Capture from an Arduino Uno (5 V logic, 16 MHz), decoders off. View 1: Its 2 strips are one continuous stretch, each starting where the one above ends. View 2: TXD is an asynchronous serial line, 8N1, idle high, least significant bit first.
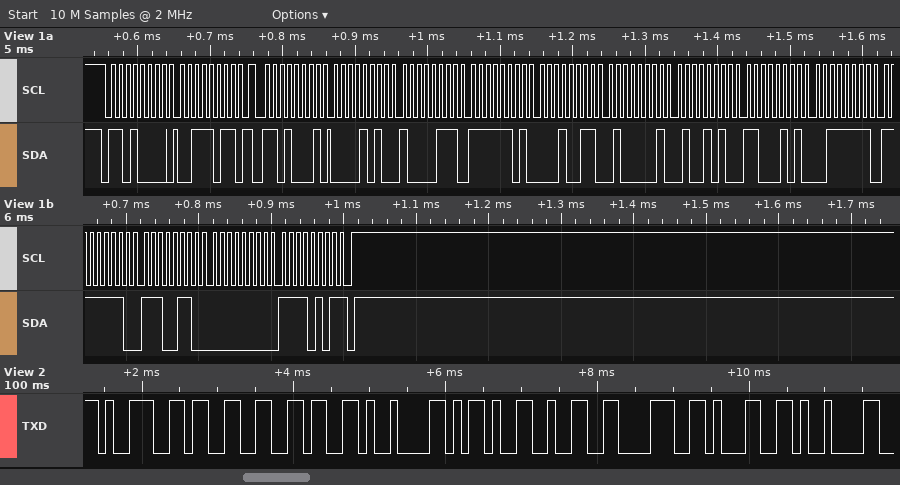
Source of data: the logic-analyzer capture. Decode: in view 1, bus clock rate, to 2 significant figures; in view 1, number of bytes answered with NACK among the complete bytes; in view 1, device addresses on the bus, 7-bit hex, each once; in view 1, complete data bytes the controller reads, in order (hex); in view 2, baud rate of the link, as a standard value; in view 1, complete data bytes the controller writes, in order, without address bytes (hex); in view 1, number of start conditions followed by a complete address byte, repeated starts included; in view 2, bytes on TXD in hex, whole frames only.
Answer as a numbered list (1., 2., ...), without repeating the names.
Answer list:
1. 100 kHz
2. 1
3. 0x68
4. 0A 87 FD 13 41 4A C5 3F FE E6 00 F5
5. 9600 baud
6. 3B
7. 2
8. 39 33 36 09 2D 32 38 31 09
